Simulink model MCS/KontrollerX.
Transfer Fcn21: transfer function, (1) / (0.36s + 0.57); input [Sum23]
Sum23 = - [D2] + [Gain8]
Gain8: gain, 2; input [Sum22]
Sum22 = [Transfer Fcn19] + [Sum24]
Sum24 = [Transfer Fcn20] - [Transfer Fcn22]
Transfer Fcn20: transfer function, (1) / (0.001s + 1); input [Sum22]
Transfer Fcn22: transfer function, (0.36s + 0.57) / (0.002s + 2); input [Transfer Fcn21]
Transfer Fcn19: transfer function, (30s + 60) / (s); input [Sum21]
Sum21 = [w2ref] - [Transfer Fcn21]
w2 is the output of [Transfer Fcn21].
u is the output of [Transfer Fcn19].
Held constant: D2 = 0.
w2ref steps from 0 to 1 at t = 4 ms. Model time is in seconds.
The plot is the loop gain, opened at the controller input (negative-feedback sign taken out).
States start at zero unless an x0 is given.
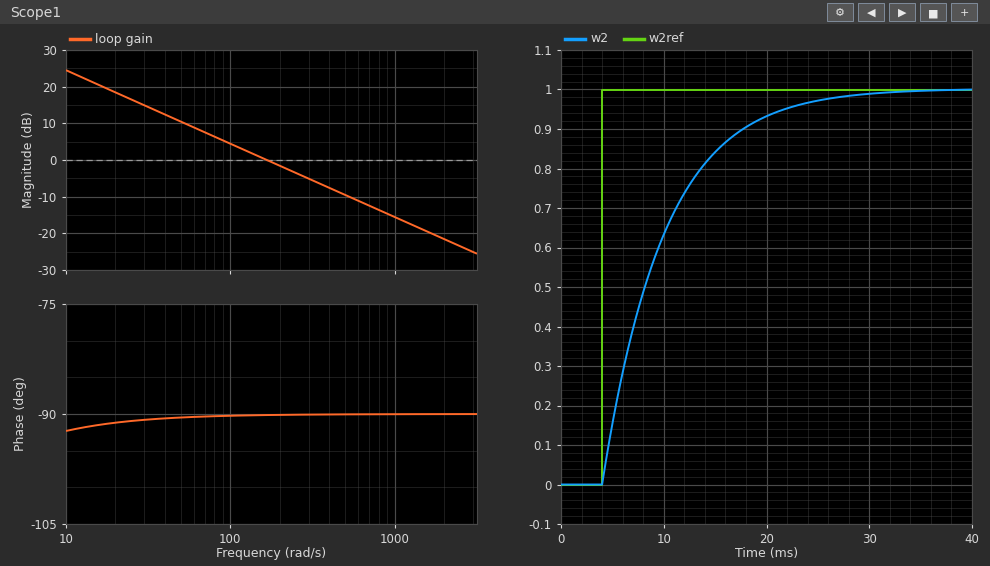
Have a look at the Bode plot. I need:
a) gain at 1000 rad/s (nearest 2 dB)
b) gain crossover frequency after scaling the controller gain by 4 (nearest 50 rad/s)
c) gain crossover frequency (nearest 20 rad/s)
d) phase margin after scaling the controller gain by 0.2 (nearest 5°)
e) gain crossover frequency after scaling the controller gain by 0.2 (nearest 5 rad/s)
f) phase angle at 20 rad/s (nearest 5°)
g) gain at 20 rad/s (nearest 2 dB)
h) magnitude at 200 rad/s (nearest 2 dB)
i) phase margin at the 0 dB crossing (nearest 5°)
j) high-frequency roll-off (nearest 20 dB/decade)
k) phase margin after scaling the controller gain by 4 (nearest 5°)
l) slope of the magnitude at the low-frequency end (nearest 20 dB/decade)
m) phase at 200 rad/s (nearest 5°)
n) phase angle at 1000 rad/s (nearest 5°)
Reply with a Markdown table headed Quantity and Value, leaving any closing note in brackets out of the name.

| Quantity | Value |
|---|---|
| gain at 1000 rad/s | -16 dB |
| gain crossover frequency after scaling the controller gain by 4 | 650 rad/s |
| gain crossover frequency | 160 rad/s |
| phase margin after scaling the controller gain by 0.2 | 90° |
| gain crossover frequency after scaling the controller gain by 0.2 | 35 rad/s |
| phase angle at 20 rad/s | -90° |
| gain at 20 rad/s | 18 dB |
| magnitude at 200 rad/s | -2 dB |
| phase margin at the 0 dB crossing | 90° |
| high-frequency roll-off | -20 dB/decade |
| phase margin after scaling the controller gain by 4 | 90° |
| slope of the magnitude at the low-frequency end | -20 dB/decade |
| phase at 200 rad/s | -90° |
| phase angle at 1000 rad/s | -90° |
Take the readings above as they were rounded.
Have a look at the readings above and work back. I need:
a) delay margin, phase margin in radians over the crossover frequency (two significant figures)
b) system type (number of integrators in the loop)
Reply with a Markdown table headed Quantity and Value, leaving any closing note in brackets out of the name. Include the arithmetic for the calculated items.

| Quantity | Value |
|---|---|
| delay margin, phase margin in radians over the crossover frequency | 90 × π / 180 / 160 = 0.0098 s |
| system type | 1 |
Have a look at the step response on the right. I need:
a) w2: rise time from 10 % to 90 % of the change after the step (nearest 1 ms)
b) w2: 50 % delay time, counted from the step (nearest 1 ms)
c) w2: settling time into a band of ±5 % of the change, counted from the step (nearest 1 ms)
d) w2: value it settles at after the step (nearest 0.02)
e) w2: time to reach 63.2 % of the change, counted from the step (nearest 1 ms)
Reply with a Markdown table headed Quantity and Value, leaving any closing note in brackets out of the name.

| Quantity | Value |
|---|---|
| w2: rise time from 10 % to 90 % of the change after the step | 13 ms |
| w2: 50 % delay time, counted from the step | 4 ms |
| w2: settling time into a band of ±5 % of the change, counted from the step | 18 ms |
| w2: value it settles at after the step | 1.00 |
| w2: time to reach 63.2 % of the change, counted from the step | 6 ms |
